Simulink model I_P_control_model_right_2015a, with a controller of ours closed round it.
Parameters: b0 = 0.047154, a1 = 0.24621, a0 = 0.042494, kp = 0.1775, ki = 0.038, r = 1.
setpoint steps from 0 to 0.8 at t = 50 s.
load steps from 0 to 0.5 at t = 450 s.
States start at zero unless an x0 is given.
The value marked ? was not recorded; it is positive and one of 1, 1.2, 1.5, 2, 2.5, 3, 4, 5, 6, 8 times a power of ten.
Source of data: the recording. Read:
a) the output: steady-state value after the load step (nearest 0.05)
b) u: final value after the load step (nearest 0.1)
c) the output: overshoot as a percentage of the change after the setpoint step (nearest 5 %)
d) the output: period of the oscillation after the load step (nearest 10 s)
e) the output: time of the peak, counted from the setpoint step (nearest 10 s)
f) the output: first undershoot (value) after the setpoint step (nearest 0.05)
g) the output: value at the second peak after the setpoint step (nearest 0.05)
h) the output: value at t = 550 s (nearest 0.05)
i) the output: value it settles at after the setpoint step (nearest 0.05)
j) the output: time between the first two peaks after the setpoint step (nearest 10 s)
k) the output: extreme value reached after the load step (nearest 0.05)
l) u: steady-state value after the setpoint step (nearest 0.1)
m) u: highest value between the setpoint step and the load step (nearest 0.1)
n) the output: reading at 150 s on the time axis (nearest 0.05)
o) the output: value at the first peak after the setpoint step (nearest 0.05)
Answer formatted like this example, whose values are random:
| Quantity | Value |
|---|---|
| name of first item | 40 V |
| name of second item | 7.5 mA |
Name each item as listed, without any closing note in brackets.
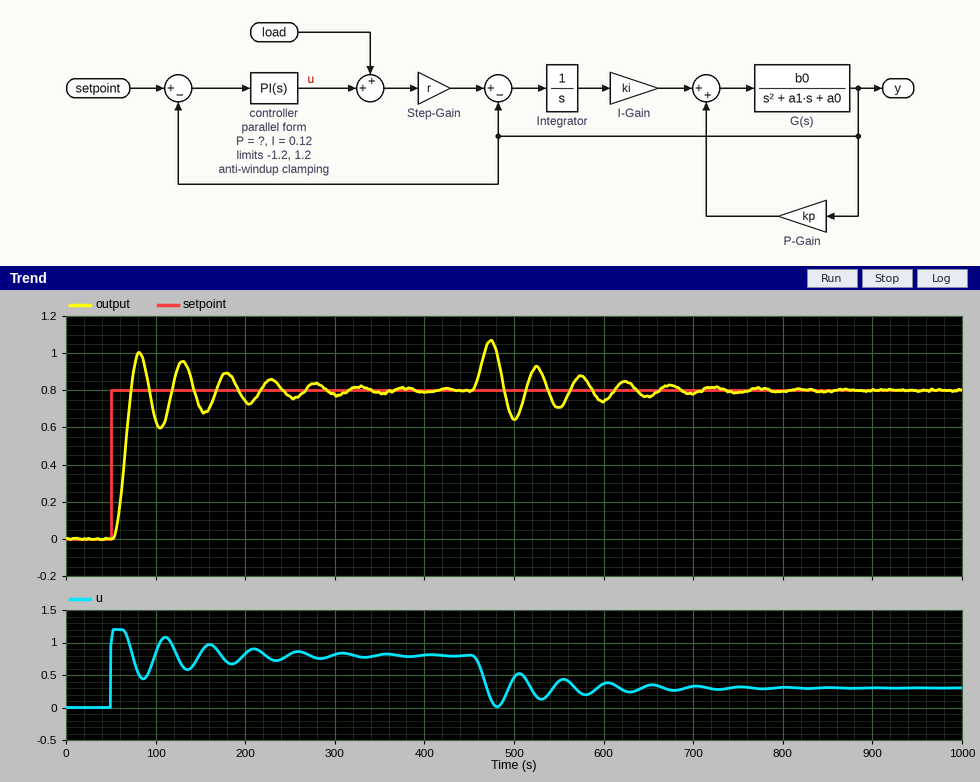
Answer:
| Quantity | Value |
|---|---|
| the output: steady-state value after the load step | 0.80 |
| u: final value after the load step | 0.3 |
| the output: overshoot as a percentage of the change after the setpoint step | 25 % |
| the output: period of the oscillation after the load step | 50 s |
| the output: time of the peak, counted from the setpoint step | 30 s |
| the output: first undershoot (value) after the setpoint step | 0.60 |
| the output: value at the second peak after the setpoint step | 0.95 |
| the output: value at t = 550 s | 0.70 |
| the output: value it settles at after the setpoint step | 0.80 |
| the output: time between the first two peaks after the setpoint step | 50 s |
| the output: extreme value reached after the load step | 1.05 |
| u: steady-state value after the setpoint step | 0.8 |
| u: highest value between the setpoint step and the load step | 1.2 |
| the output: reading at 150 s on the time axis | 0.70 |
| the output: value at the first peak after the setpoint step | 1.00 |
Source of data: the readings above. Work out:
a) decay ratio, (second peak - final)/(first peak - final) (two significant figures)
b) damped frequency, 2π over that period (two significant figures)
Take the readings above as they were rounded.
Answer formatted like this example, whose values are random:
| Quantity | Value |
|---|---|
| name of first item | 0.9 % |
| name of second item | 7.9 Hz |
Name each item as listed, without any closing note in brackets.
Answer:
| Quantity | Value |
|---|---|
| decay ratio, (second peak - final)/(first peak - final) | 0.75 |
| damped frequency, 2π over that period | 0.13 rad/s |
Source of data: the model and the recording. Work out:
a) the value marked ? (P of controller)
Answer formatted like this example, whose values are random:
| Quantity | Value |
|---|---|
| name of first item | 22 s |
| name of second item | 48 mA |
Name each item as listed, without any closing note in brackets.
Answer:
| Quantity | Value |
|---|---|
| the value marked ? | 1.2 |
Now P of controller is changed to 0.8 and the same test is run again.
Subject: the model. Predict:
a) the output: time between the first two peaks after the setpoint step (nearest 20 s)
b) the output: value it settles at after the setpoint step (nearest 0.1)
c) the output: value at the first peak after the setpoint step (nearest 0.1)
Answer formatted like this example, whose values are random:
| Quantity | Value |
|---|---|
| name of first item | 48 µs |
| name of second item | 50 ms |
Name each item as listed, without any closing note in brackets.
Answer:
| Quantity | Value |
|---|---|
| the output: time between the first two peaks after the setpoint step | 60 s |
| the output: value it settles at after the setpoint step | 0.8 |
| the output: value at the first peak after the setpoint step | 1.1 |
